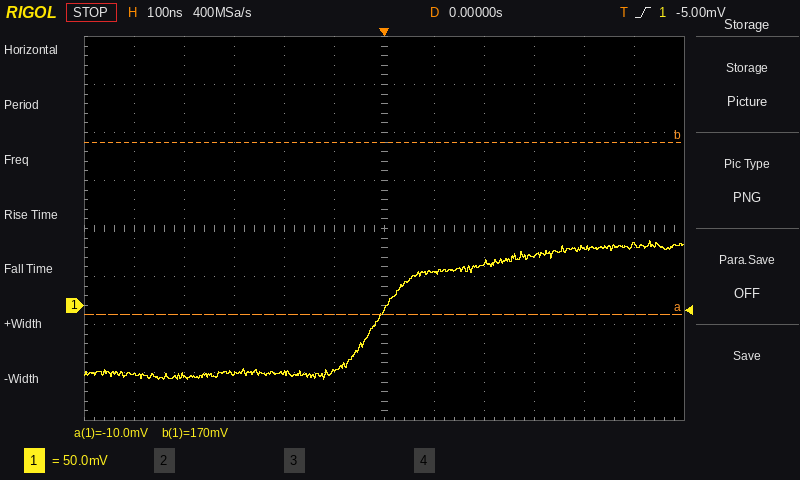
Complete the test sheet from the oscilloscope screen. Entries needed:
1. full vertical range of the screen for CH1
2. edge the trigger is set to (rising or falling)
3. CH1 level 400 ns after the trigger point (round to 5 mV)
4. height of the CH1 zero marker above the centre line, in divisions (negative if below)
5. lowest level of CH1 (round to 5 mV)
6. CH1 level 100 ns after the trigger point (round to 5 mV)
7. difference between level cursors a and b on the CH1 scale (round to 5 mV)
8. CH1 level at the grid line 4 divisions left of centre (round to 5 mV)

400 mV
rising
60 mV
-1.6 div
-75 mV
35 mV
180 mV
-75 mV
